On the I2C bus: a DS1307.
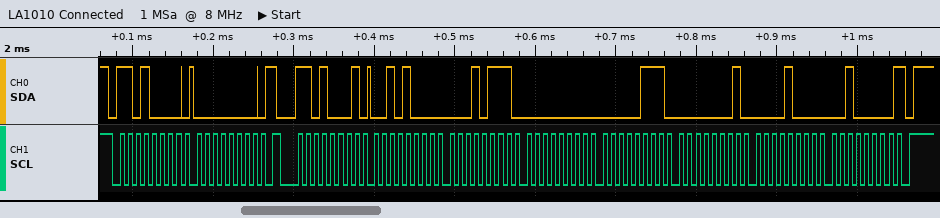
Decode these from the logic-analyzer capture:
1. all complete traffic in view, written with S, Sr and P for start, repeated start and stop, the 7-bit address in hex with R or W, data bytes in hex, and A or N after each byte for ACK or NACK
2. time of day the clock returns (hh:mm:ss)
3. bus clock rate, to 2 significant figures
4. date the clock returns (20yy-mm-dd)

S 68W A 00 A Sr 68R A 28 A 17 A 00 A 07 A 01 A 08 A 20 N P
00:17:28
100 kHz
2020-08-01
